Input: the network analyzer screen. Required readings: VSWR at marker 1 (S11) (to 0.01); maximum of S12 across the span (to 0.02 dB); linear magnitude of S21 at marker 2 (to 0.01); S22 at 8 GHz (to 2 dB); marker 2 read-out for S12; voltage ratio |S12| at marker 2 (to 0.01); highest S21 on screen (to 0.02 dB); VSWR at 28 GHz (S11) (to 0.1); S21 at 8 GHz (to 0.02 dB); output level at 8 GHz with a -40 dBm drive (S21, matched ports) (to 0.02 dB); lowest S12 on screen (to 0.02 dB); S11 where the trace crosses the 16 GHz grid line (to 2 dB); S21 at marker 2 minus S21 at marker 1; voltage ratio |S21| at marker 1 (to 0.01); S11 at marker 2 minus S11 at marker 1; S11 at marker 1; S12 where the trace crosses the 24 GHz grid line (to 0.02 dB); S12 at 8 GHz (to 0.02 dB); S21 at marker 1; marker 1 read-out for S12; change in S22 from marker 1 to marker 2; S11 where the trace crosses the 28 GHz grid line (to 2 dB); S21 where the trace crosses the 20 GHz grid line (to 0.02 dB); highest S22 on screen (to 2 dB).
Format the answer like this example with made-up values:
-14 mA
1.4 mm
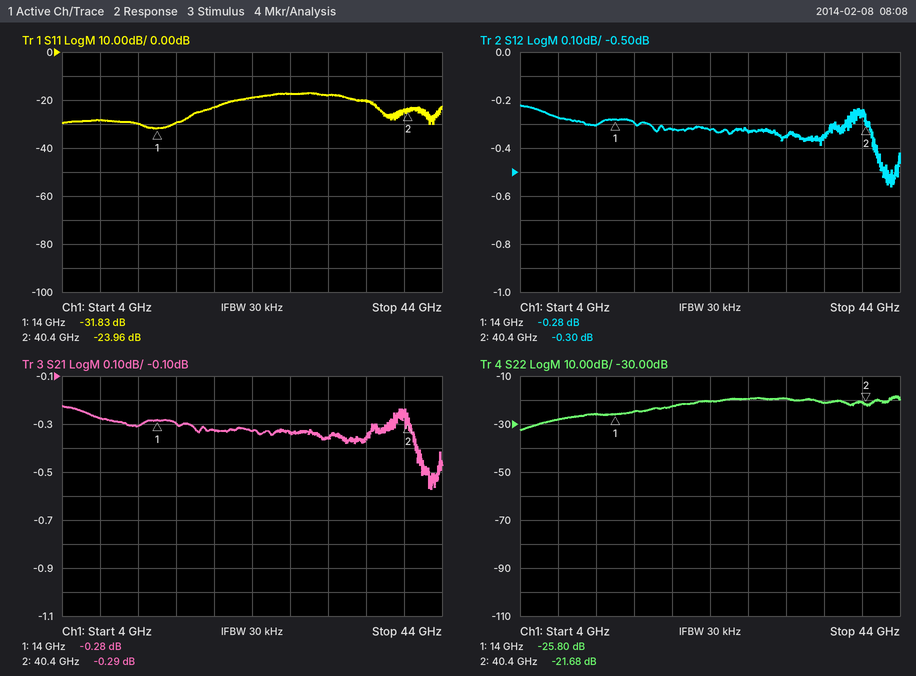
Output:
1.05
-0.22 dB
0.97
-28 dB
-0.30 dB
0.97
-0.22 dB
1.3
-0.28 dB
-40.28 dBm
-0.56 dB
-30 dB
-0.01 dB
0.97
7.87 dB
-31.83 dB
-0.32 dB
-0.28 dB
-0.28 dB
-0.28 dB
4.12 dB
-18 dB
-0.32 dB
-18 dB
